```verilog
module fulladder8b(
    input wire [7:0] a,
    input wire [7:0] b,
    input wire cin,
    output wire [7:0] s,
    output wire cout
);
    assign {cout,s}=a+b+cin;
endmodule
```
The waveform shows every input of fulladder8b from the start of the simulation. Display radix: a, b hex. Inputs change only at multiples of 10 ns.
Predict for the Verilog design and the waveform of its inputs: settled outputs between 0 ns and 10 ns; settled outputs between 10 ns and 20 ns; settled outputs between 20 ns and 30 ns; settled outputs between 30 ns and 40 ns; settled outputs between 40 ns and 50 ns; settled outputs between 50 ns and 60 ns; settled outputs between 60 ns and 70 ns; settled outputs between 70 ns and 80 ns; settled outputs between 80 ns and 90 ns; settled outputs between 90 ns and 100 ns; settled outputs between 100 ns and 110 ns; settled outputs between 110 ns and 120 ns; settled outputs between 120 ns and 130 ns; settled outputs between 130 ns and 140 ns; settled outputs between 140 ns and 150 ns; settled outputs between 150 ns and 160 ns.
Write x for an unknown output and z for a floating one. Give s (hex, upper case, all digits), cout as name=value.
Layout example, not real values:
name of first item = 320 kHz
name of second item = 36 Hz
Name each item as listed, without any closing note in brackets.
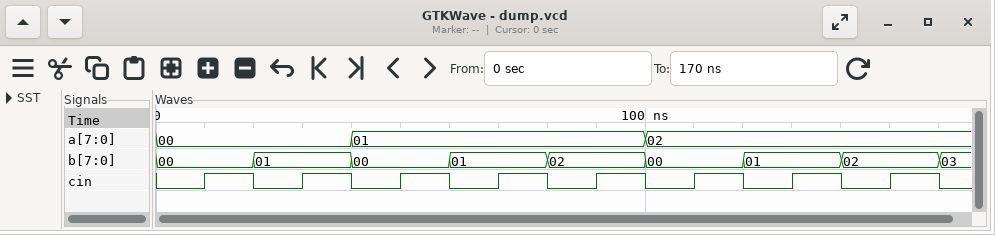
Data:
settled outputs between 0 ns and 10 ns = s=00, cout=0
settled outputs between 10 ns and 20 ns = s=01, cout=0
settled outputs between 20 ns and 30 ns = s=01, cout=0
settled outputs between 30 ns and 40 ns = s=02, cout=0
settled outputs between 40 ns and 50 ns = s=01, cout=0
settled outputs between 50 ns and 60 ns = s=02, cout=0
settled outputs between 60 ns and 70 ns = s=02, cout=0
settled outputs between 70 ns and 80 ns = s=03, cout=0
settled outputs between 80 ns and 90 ns = s=03, cout=0
settled outputs between 90 ns and 100 ns = s=04, cout=0
settled outputs between 100 ns and 110 ns = s=02, cout=0
settled outputs between 110 ns and 120 ns = s=03, cout=0
settled outputs between 120 ns and 130 ns = s=03, cout=0
settled outputs between 130 ns and 140 ns = s=04, cout=0
settled outputs between 140 ns and 150 ns = s=04, cout=0
settled outputs between 150 ns and 160 ns = s=05, cout=0
